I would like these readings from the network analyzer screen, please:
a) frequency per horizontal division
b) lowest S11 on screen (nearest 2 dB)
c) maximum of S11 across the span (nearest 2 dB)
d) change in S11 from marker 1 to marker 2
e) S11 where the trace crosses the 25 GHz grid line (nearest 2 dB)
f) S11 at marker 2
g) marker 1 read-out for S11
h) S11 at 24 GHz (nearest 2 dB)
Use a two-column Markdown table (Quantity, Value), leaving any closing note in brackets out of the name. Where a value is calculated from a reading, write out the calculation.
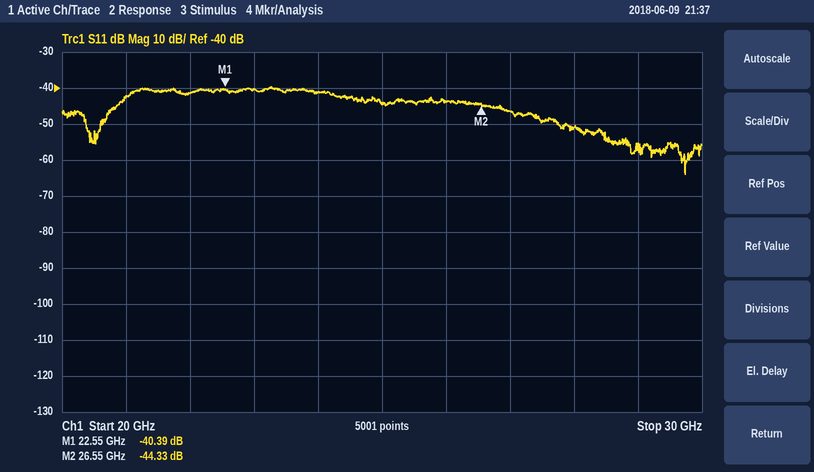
| Quantity | Value |
|---|---|
| frequency per horizontal division | 1 GHz |
| lowest S11 on screen | -64 dB |
| maximum of S11 across the span | -40 dB |
| change in S11 from marker 1 to marker 2 | -44.33 − (-40.39) = -3.94 dB |
| S11 where the trace crosses the 25 GHz grid line | -44 dB |
| S11 at marker 2 | -44.33 dB |
| marker 1 read-out for S11 | -40.39 dB |
| S11 at 24 GHz | -42 dB |
